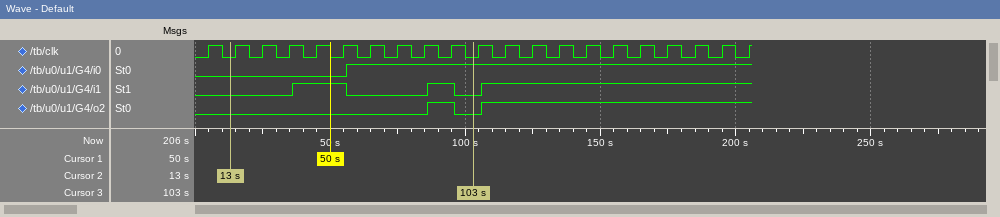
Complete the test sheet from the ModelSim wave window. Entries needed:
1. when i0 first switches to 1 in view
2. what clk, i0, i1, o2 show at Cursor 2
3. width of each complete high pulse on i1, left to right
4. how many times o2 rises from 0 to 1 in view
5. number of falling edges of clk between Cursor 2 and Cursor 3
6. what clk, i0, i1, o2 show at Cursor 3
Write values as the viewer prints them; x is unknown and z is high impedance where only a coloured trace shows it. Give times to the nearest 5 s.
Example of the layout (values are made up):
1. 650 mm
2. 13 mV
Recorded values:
1. 55 s
2. clk=0, i0=0, i1=0, o2=0
3. 20 s, 10 s
4. 2
5. 9
6. clk=0, i0=1, i1=0, o2=0
